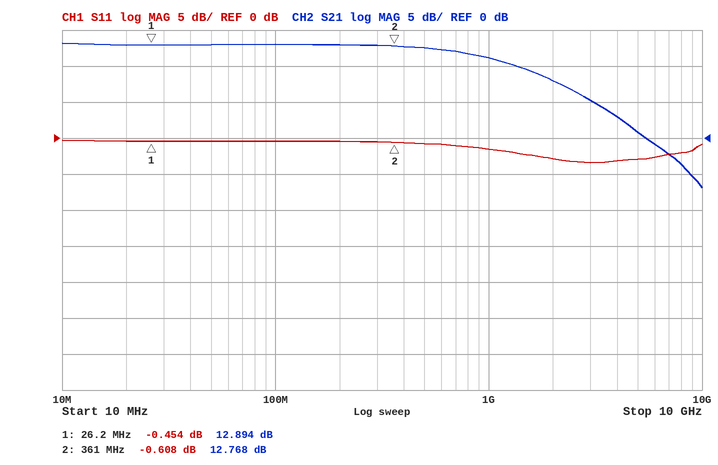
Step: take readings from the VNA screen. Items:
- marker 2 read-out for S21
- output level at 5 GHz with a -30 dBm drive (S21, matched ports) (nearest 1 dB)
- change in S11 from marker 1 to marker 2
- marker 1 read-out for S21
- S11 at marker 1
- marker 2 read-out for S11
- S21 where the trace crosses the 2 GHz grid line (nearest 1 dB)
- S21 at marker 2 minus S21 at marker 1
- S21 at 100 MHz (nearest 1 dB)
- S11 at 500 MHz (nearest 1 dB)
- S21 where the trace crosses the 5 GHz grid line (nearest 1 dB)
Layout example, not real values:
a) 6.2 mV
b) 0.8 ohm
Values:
a) 12.768 dB
b) -29 dBm
c) -0.154 dB
d) 12.894 dB
e) -0.454 dB
f) -0.608 dB
g) 8 dB
h) -0.126 dB
i) 13 dB
j) -1 dB
k) 1 dB
